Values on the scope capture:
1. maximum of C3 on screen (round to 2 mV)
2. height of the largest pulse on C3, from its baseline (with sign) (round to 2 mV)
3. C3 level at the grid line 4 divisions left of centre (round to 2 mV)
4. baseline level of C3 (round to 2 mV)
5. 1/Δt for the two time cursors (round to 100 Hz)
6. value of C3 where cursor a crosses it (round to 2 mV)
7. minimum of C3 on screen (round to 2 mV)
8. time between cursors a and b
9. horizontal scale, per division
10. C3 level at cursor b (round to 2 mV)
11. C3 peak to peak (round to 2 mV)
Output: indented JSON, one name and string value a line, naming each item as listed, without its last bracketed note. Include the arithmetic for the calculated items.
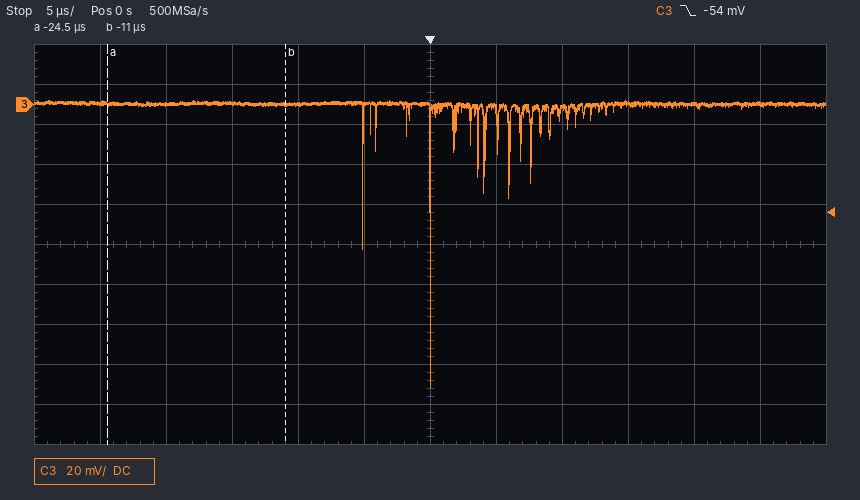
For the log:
{
  "maximum of C3 on screen": "2 mV",
  "height of the largest pulse on C3, from its baseline (with sign)": "-142 mV − (0 mV) = -142 mV",
  "C3 level at the grid line 4 divisions left of centre": "0 mV",
  "baseline level of C3": "0 mV",
  "1/Δt for the two time cursors": "1 / 13.5 µs ≈ 74.1 kHz",
  "value of C3 where cursor a crosses it": "0 mV",
  "minimum of C3 on screen": "-142 mV",
  "time between cursors a and b": "-11 µs − (-24.5 µs) = 13.5 µs",
  "horizontal scale, per division": "5 µs",
  "C3 level at cursor b": "0 mV",
  "C3 peak to peak": "2 mV − (-142 mV) = 144 mV"
}
